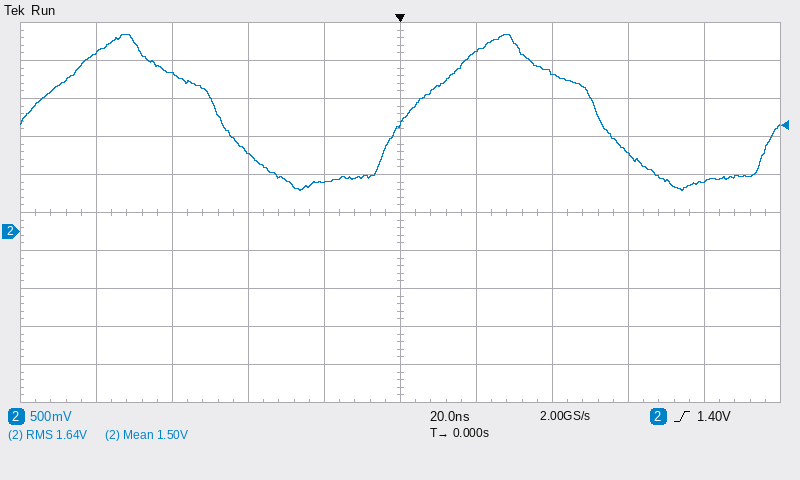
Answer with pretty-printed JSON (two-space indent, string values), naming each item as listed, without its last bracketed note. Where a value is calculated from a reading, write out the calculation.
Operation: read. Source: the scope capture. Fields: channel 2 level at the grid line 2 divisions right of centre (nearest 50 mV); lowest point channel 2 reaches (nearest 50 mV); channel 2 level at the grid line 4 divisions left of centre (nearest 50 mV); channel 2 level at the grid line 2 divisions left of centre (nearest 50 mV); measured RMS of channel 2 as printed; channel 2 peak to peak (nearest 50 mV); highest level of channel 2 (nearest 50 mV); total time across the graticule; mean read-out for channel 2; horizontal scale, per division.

{
  "channel 2 level at the grid line 2 divisions right of centre": "2.10 V",
  "lowest point channel 2 reaches": "550 mV",
  "channel 2 level at the grid line 4 divisions left of centre": "2.35 V",
  "channel 2 level at the grid line 2 divisions left of centre": "1.05 V",
  "measured RMS of channel 2 as printed": "1.64 V",
  "channel 2 peak to peak": "2.60 V − (550 mV) = 2.05 V",
  "highest level of channel 2": "2.60 V",
  "total time across the graticule": "200 ns",
  "mean read-out for channel 2": "1.50 V",
  "horizontal scale, per division": "20 ns"
}
